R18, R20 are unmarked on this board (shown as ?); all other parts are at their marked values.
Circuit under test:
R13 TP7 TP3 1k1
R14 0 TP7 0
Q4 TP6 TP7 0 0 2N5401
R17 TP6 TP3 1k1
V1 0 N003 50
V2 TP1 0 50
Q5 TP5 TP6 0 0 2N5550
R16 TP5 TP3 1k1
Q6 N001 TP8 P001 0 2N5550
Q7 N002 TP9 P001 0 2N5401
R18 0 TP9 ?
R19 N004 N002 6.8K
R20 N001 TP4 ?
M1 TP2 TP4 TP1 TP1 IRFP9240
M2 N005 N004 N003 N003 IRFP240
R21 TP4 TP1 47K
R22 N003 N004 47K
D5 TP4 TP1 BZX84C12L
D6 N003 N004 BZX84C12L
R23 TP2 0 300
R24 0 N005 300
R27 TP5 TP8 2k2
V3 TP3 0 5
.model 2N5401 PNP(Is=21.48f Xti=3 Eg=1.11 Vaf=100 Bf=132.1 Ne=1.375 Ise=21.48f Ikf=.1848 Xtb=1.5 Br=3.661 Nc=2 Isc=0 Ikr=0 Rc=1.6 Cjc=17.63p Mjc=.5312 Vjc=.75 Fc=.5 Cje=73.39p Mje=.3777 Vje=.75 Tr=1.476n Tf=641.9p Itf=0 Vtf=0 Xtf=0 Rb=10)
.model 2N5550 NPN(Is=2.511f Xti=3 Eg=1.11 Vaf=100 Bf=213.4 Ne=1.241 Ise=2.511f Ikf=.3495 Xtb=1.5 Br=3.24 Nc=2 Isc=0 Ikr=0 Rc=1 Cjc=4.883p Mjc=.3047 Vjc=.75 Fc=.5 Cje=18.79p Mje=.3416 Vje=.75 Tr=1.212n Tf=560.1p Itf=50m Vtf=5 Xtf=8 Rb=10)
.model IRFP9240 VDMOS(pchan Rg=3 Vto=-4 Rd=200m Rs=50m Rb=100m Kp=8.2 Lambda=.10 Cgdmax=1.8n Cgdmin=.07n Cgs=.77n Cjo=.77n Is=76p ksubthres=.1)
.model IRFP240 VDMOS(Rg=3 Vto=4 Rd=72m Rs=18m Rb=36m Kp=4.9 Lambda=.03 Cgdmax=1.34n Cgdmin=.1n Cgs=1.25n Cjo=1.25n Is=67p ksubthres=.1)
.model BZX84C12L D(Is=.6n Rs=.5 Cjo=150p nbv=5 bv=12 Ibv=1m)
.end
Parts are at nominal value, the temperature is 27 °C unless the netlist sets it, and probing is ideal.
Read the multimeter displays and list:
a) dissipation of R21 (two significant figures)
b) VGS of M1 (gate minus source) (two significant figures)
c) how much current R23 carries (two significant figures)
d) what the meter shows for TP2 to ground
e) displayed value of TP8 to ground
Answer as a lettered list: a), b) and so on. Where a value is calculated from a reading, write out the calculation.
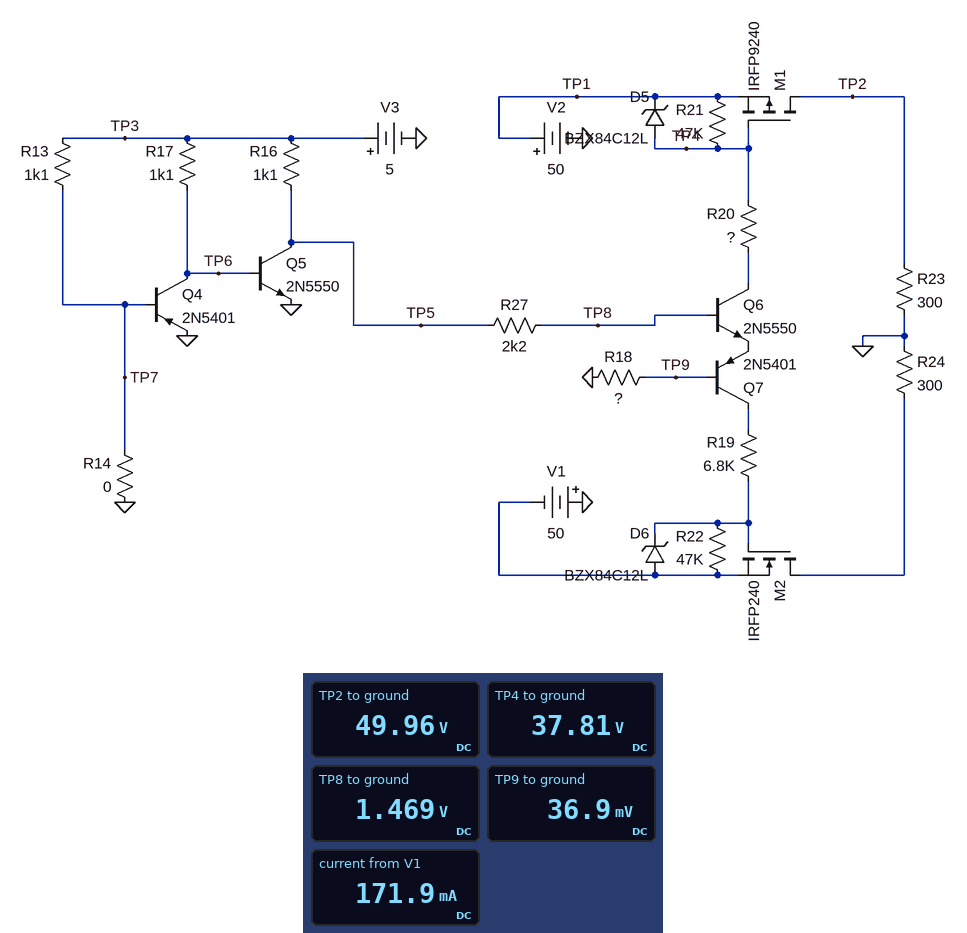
a) (50 V - 37.81 V)^2 / 47 kΩ = 3.2 mW
b) 37.81 V - 50 V = -12 V
c) (49.96 V) / 300 Ω = 170 mA
d) 49.96 V
e) 1.469 V
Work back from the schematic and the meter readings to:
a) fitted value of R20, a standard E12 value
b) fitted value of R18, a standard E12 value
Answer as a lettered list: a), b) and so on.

a) 8.2 kΩ
b) 820 Ω
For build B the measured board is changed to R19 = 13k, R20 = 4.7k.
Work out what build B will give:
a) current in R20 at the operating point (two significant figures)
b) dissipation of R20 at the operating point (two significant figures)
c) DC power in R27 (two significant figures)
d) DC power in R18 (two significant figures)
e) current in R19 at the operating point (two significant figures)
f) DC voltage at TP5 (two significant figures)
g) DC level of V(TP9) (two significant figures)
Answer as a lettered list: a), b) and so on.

a) 6.3 mA
b) 190 mW
c) 6.2 µW
d) 8.4 mW
e) 3.2 mA
f) 4.2 V
g) 2.6 V
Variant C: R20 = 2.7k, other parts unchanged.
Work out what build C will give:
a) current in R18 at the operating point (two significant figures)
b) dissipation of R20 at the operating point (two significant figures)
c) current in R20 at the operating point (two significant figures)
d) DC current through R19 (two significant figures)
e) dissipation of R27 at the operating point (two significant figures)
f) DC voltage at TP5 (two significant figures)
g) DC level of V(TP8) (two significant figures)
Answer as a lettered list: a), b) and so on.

a) 3.1 mA
b) 220 mW
c) 9.1 mA
d) 6.0 mA
e) 11 µW
f) 4.2 V
g) 4.0 V
